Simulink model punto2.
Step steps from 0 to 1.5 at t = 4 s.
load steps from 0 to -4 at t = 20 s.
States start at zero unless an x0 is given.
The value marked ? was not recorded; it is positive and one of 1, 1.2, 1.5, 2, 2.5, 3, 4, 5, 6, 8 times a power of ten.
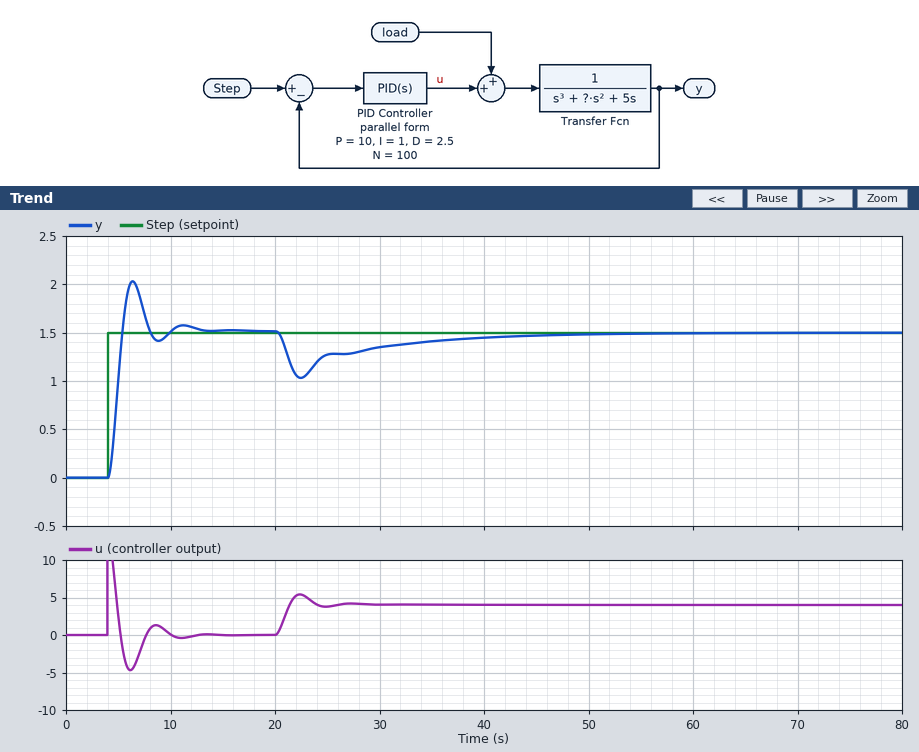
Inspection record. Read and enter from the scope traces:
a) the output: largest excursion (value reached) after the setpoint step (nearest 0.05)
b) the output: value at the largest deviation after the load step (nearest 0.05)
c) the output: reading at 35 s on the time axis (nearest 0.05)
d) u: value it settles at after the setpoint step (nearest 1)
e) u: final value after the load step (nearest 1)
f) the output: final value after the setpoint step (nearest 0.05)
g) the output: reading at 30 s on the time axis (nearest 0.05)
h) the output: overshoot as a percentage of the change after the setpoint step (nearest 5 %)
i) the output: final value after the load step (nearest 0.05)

2.05
1.05
1.40
0
4
1.50
1.35
35 %
1.50
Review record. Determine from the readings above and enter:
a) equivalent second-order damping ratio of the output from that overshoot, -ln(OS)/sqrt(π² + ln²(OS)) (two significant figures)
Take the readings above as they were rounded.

0.32
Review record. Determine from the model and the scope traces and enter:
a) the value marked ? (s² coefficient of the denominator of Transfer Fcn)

6
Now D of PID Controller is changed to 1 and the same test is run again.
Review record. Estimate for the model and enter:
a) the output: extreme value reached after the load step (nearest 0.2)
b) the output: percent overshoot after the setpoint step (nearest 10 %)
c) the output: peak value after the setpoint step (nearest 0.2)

1.0
50 %
2.2
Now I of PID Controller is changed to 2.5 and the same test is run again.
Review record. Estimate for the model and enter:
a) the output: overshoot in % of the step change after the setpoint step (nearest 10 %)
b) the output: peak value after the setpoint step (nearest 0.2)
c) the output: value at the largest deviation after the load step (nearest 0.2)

50 %
2.2
1.0
